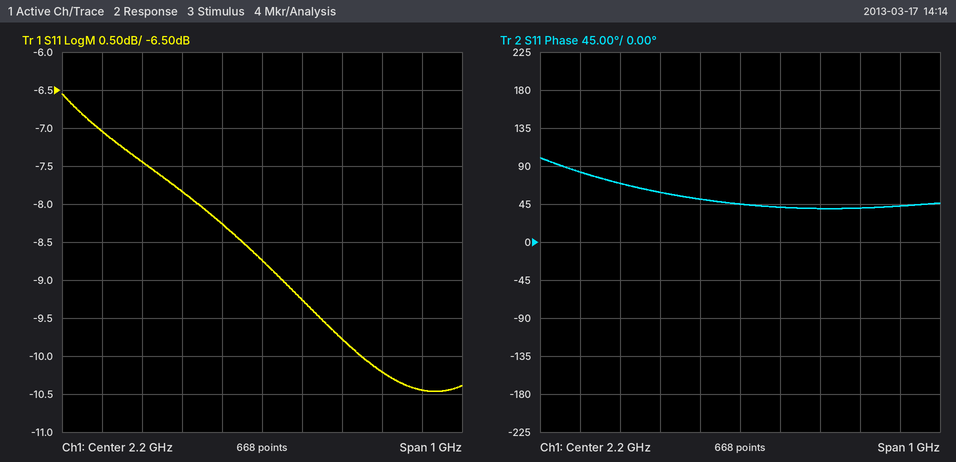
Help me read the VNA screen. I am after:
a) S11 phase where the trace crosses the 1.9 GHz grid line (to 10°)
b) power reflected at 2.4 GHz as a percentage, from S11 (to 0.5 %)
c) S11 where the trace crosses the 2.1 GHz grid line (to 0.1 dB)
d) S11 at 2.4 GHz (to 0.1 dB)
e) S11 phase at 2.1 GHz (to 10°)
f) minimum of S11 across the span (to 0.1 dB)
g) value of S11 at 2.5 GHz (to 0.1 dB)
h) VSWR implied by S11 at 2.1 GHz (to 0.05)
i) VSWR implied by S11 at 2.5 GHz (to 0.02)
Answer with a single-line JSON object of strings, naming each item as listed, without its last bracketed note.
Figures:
{"S11 phase where the trace crosses the 1.9 GHz grid line": "70°", "power reflected at 2.4 GHz as a percentage, from S11": "10.5 %", "S11 where the trace crosses the 2.1 GHz grid line": "-8.3 dB", "S11 at 2.4 GHz": "-9.8 dB", "S11 phase at 2.1 GHz": "50°", "minimum of S11 across the span": "-10.5 dB", "value of S11 at 2.5 GHz": "-10.2 dB", "VSWR implied by S11 at 2.1 GHz": "2.25", "VSWR implied by S11 at 2.5 GHz": "1.90"}
